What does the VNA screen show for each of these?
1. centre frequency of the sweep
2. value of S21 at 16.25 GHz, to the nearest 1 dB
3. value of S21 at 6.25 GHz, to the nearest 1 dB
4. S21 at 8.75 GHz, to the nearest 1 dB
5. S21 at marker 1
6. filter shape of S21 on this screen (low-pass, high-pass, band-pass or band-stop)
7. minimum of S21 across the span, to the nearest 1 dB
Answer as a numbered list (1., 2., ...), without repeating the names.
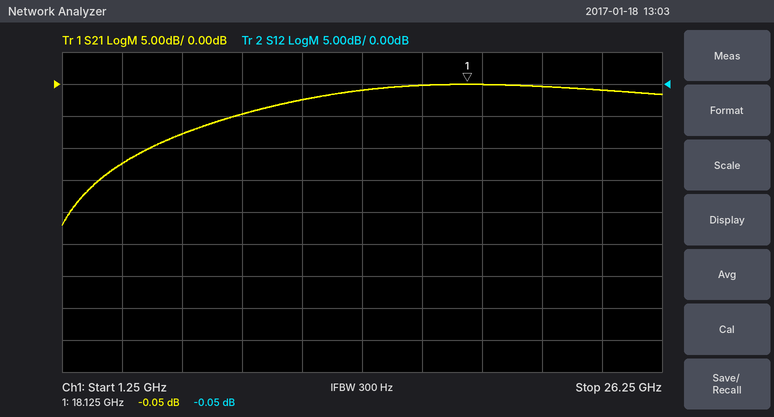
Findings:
1. 13.75 GHz
2. 0 dB
3. -8 dB
4. -5 dB
5. -0.05 dB
6. high-pass
7. -22 dB
